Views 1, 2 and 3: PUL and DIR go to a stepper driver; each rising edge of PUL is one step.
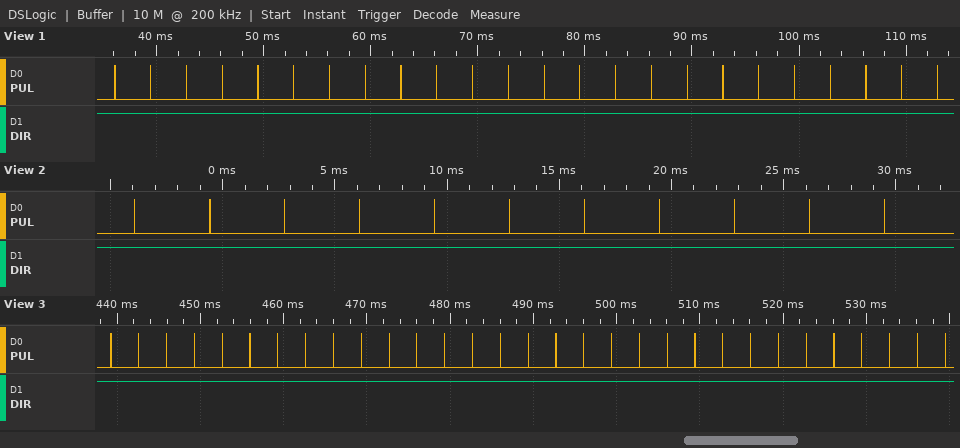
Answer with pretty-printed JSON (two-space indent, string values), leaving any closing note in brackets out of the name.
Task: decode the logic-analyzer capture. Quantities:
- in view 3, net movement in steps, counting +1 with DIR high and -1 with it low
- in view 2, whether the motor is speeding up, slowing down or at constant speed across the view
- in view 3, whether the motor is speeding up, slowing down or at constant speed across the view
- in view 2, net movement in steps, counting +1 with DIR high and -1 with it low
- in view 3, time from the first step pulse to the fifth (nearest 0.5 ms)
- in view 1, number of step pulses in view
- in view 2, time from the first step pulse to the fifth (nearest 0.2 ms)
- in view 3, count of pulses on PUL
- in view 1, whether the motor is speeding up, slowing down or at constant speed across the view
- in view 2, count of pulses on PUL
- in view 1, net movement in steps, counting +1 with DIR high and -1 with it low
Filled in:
{
  "in view 3, net movement in steps, counting +1 with DIR high and -1 with it low": "+31",
  "in view 2, whether the motor is speeding up, slowing down or at constant speed across the view": "constant speed",
  "in view 3, whether the motor is speeding up, slowing down or at constant speed across the view": "constant speed",
  "in view 2, net movement in steps, counting +1 with DIR high and -1 with it low": "+11",
  "in view 3, time from the first step pulse to the fifth": "13.5 ms",
  "in view 1, number of step pulses in view": "24",
  "in view 2, time from the first step pulse to the fifth": "13.4 ms",
  "in view 3, count of pulses on PUL": "31",
  "in view 1, whether the motor is speeding up, slowing down or at constant speed across the view": "constant speed",
  "in view 2, count of pulses on PUL": "11",
  "in view 1, net movement in steps, counting +1 with DIR high and -1 with it low": "+24"
}
